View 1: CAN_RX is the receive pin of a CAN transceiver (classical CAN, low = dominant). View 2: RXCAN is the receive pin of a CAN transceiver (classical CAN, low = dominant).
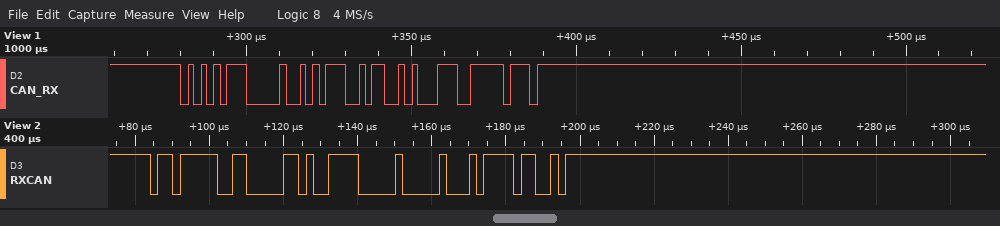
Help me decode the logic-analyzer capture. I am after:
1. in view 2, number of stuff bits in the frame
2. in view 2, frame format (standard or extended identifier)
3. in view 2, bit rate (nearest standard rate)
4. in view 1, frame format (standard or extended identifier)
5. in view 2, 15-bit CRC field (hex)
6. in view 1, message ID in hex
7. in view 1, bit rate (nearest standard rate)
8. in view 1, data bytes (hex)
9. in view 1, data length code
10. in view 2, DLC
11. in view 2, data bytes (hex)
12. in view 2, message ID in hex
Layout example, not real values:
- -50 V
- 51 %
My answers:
- 4
- standard
- 500 kbit/s
- standard
- 0x05EC
- 0x55C
- 500 kbit/s
- B9 65
- 2
- 2
- 9E 00
- 0x6FB
